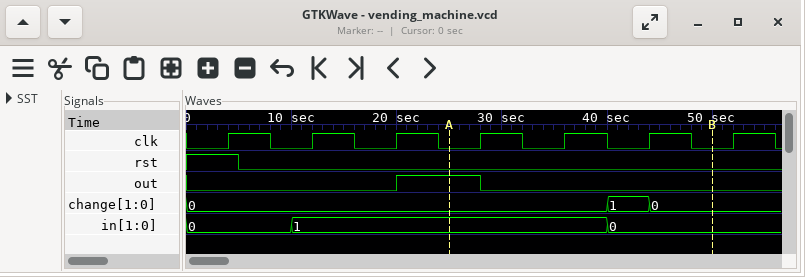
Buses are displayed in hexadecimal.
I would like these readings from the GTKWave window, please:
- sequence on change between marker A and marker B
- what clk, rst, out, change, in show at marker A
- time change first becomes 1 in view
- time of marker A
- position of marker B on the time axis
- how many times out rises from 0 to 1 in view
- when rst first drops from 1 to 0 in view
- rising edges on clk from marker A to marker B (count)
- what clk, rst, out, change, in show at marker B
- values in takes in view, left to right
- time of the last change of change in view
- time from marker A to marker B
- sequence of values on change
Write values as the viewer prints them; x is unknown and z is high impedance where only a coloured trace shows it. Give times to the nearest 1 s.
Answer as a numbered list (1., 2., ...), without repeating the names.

1. 0, 1, 0
2. clk=0, rst=0, out=1, change=0, in=1
3. 40 s
4. 25 s
5. 50 s
6. 1
7. 5 s
8. 3
9. clk=0, rst=0, out=0, change=0, in=0
10. 0, 1, 0
11. 44 s
12. 25 s
13. 0, 1, 0
